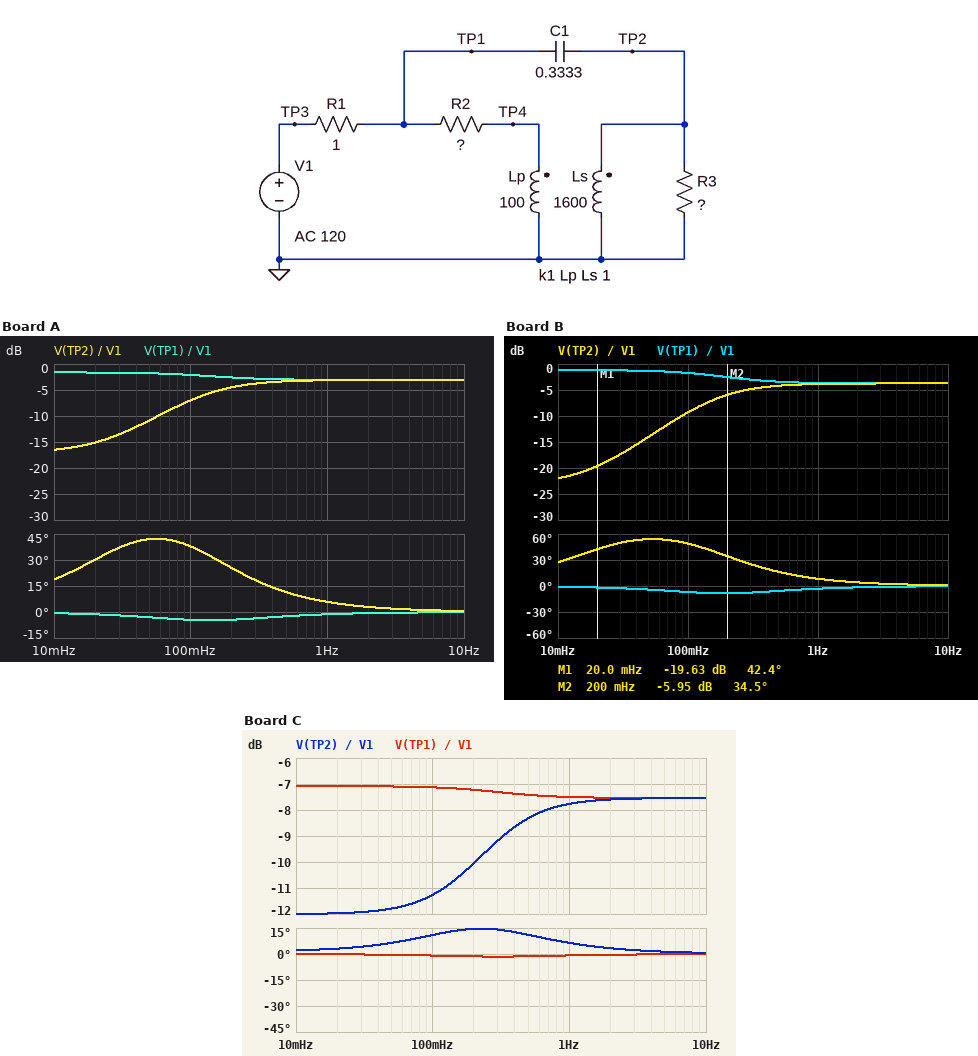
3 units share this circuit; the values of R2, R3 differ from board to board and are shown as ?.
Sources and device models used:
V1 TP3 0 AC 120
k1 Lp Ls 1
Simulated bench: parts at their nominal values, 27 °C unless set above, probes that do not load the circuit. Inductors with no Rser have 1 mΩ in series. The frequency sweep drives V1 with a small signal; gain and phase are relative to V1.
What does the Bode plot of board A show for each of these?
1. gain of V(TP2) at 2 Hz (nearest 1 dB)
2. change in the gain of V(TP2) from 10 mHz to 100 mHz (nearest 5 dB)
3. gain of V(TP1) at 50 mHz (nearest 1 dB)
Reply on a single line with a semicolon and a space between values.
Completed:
-3 dB; 10 dB; -2 dB
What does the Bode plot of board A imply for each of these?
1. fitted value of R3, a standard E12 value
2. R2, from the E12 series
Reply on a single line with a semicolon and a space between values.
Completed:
3.3 Ω; 4.7 Ω
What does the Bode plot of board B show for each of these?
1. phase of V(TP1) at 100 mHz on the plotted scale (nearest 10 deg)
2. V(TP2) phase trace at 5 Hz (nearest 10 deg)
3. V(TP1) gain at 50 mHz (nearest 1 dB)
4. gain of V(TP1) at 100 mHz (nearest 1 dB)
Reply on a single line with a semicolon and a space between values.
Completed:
-10 deg; 0 deg; -1 dB; -2 dB
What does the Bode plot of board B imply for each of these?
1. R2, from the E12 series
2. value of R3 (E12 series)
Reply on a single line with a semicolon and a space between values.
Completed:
6.8 Ω; 2.2 Ω
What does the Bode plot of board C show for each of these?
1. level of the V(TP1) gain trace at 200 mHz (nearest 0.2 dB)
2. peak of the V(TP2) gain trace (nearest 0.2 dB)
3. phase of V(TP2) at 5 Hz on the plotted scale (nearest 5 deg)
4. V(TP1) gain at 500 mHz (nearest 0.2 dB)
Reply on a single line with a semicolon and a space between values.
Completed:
-7.2 dB; -7.6 dB; 0 deg; -7.4 dB
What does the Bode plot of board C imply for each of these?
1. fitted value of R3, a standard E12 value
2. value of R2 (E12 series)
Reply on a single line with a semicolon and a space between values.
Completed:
1.8 Ω; 0.68 Ω
